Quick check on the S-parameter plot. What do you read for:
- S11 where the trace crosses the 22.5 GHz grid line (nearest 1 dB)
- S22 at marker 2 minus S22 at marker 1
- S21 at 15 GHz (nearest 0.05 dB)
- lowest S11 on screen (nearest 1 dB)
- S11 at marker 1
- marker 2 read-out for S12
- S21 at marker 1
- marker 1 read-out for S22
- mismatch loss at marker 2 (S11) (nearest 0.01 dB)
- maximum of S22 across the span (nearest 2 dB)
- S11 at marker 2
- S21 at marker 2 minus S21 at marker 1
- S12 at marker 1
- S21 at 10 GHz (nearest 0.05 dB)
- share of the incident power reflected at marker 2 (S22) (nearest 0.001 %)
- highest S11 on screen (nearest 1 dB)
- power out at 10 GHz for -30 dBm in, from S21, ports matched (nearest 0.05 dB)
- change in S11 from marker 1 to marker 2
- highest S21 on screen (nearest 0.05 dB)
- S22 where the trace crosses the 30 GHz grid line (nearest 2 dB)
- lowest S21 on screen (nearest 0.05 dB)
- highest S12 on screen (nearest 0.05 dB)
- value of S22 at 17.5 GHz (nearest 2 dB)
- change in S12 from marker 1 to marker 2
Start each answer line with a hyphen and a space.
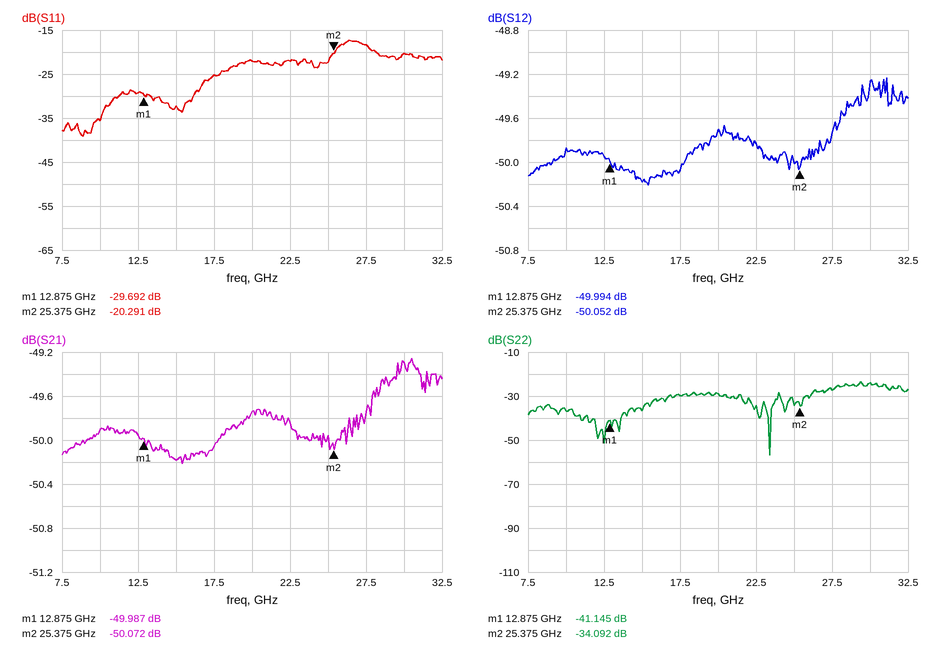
- -22 dB
- 7.053 dB
- -50.20 dB
- -39 dB
- -29.692 dB
- -50.052 dB
- -49.987 dB
- -41.145 dB
- 0.04 dB
- -24 dB
- -20.291 dB
- -0.085 dB
- -49.994 dB
- -49.90 dB
- 0.039 %
- -17 dB
- -79.90 dBm
- 9.401 dB
- -49.25 dB
- -24 dB
- -50.20 dB
- -49.25 dB
- -30 dB
- -0.058 dB
